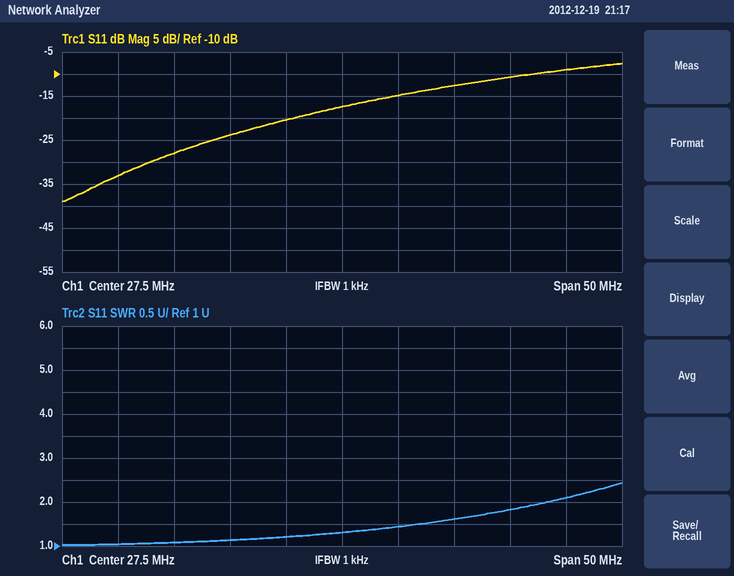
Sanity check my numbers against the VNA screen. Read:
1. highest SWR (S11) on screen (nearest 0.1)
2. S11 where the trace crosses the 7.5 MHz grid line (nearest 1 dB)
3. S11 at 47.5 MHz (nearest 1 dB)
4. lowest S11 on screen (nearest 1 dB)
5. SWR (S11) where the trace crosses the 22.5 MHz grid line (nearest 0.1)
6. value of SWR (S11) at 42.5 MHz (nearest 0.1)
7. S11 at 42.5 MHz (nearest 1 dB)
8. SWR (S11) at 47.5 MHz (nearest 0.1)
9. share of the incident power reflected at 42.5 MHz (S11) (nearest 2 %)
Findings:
2.4
-33 dB
-9 dB
-39 dB
1.2
1.8
-11 dB
2.1
8 %
